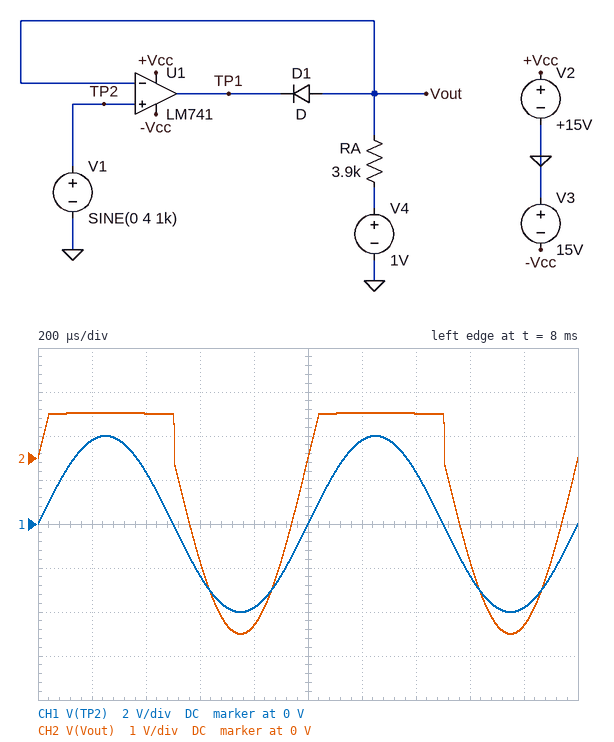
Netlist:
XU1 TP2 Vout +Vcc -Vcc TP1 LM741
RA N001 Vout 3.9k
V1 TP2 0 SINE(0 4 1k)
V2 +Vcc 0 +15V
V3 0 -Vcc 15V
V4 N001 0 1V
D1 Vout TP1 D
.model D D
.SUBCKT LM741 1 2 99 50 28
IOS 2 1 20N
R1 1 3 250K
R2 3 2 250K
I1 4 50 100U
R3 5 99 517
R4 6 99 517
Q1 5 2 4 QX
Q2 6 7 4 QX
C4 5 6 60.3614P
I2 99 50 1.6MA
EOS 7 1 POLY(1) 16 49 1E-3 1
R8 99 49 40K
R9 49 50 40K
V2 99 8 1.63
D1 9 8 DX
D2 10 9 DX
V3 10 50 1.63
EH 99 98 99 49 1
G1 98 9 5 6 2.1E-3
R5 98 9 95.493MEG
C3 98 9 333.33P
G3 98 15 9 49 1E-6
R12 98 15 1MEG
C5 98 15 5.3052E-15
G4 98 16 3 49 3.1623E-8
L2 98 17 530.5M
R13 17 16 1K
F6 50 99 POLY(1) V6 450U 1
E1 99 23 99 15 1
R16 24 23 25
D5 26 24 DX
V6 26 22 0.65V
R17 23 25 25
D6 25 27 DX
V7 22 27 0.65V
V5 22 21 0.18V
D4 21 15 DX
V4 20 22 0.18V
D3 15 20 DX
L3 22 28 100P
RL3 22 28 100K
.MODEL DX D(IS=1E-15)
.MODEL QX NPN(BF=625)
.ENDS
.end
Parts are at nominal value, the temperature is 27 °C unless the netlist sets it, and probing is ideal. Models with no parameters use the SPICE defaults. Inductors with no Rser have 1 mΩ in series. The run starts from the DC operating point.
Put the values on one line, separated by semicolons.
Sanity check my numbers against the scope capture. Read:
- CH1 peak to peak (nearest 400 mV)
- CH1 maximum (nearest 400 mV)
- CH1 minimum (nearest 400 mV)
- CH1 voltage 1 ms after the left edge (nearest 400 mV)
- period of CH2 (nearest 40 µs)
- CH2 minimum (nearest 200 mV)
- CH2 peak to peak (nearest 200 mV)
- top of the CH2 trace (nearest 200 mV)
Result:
8.0 V; 4.0 V; -4.0 V; 0 V; 1.00 ms; -4.0 V; 5.0 V; 1.0 V
